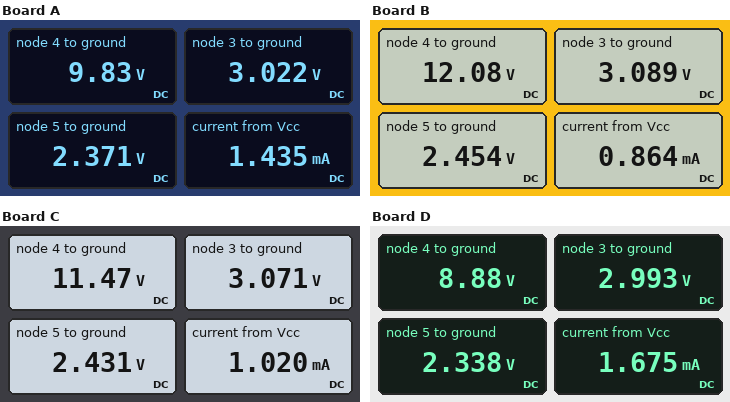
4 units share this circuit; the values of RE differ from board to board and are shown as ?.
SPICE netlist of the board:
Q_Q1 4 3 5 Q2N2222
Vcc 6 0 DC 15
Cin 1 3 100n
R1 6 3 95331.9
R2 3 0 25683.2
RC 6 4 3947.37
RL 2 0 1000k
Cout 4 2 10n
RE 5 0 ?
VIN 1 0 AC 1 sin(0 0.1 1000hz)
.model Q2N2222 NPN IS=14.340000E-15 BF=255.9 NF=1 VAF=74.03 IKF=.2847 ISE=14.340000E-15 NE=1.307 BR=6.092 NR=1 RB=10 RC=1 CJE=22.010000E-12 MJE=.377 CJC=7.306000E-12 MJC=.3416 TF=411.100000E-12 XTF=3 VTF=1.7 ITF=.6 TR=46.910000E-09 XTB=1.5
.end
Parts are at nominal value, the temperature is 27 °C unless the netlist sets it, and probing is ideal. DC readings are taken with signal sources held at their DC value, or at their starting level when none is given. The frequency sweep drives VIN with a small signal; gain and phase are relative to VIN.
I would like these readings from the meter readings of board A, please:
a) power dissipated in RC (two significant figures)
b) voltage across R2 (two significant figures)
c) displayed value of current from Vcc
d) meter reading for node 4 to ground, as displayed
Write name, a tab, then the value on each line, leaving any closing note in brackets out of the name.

power dissipated in RC	6.8 mW
voltage across R2	3.0 V
displayed value of current from Vcc	1.435 mA
meter reading for node 4 to ground, as displayed	9.83 V
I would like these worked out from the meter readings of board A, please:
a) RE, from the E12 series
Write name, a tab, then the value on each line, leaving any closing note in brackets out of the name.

RE, from the E12 series	1.8 kΩ
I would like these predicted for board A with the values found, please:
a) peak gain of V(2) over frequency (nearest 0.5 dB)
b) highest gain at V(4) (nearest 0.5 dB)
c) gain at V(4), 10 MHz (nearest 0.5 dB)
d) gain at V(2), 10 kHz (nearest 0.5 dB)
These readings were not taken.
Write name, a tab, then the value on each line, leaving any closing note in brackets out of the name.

peak gain of V(2) over frequency	6.5 dB
highest gain at V(4)	6.5 dB
gain at V(4), 10 MHz	5.0 dB
gain at V(2), 10 kHz	6.5 dB
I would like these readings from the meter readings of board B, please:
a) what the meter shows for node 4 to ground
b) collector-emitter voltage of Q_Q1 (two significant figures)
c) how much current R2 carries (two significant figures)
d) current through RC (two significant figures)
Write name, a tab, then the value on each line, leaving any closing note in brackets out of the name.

what the meter shows for node 4 to ground	12.08 V
collector-emitter voltage of Q_Q1	9.6 V
how much current R2 carries	120 µA
current through RC	740 µA
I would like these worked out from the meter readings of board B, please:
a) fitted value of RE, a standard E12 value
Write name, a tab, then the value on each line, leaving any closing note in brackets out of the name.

fitted value of RE, a standard E12 value	3.3 kΩ
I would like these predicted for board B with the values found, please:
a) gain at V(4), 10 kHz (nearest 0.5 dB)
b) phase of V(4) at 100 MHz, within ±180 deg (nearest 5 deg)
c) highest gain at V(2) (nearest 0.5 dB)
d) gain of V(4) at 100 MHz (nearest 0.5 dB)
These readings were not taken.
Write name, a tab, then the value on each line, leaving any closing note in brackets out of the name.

gain at V(4), 10 kHz	1.5 dB
phase of V(4) at 100 MHz, within ±180 deg	10 deg
highest gain at V(2)	1.5 dB
gain of V(4) at 100 MHz	0.5 dB
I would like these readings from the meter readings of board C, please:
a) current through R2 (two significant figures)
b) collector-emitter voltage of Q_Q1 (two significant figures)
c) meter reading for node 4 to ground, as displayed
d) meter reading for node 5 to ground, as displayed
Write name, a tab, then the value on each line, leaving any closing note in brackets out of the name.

current through R2	120 µA
collector-emitter voltage of Q_Q1	9.0 V
meter reading for node 4 to ground, as displayed	11.47 V
meter reading for node 5 to ground, as displayed	2.431 V
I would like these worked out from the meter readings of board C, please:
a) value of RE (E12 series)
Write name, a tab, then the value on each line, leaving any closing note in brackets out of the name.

value of RE	2.7 kΩ
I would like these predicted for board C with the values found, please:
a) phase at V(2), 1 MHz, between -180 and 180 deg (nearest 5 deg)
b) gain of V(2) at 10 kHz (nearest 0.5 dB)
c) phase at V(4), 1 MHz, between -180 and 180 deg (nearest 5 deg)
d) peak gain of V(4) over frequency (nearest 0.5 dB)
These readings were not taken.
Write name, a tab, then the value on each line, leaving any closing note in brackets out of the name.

phase at V(2), 1 MHz, between -180 and 180 deg	170 deg
gain of V(2) at 10 kHz	3.0 dB
phase at V(4), 1 MHz, between -180 and 180 deg	170 deg
peak gain of V(4) over frequency	3.0 dB
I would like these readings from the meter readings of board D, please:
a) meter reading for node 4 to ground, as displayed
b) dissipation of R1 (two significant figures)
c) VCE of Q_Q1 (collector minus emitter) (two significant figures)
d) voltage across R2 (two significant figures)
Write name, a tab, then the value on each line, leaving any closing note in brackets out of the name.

meter reading for node 4 to ground, as displayed	8.88 V
dissipation of R1	1.5 mW
VCE of Q_Q1 (collector minus emitter)	6.5 V
voltage across R2	3.0 V
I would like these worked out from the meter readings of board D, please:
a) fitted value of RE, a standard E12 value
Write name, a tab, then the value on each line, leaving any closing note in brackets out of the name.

fitted value of RE, a standard E12 value	1.5 kΩ
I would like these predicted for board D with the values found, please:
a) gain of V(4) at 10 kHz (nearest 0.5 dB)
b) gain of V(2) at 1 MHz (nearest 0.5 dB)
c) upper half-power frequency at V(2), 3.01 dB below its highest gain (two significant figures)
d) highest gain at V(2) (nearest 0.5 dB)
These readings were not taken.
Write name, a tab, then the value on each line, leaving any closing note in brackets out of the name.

gain of V(4) at 10 kHz	8.0 dB
gain of V(2) at 1 MHz	8.0 dB
upper half-power frequency at V(2), 3.01 dB below its highest gain	15 MHz
highest gain at V(2)	8.0 dB
